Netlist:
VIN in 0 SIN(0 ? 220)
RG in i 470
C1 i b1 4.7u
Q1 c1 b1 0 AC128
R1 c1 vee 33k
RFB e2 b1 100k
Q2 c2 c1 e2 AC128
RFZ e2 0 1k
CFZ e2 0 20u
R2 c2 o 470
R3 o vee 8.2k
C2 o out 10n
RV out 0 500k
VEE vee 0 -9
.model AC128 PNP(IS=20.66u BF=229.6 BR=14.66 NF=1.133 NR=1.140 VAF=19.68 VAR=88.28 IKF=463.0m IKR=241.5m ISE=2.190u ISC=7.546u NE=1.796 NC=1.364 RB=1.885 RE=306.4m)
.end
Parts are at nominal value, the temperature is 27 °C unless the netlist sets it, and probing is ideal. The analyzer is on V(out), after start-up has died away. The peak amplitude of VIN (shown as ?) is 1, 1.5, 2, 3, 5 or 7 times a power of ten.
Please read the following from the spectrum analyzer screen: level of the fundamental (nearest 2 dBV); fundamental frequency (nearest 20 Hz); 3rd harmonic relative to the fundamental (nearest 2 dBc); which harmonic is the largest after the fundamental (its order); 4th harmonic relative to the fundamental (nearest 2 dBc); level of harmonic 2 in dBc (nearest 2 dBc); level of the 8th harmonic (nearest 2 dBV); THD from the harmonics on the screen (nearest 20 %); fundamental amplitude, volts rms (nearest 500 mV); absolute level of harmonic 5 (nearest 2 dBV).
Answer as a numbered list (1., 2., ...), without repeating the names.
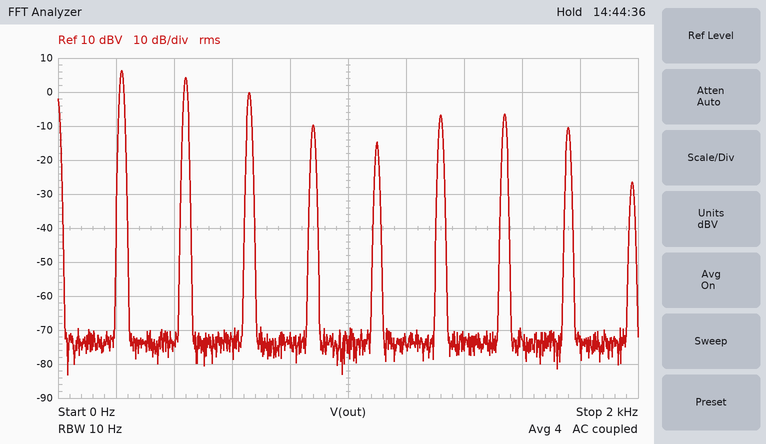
1. 6 dBV
2. 220 Hz
3. -6 dBc
4. 2
5. -16 dBc
6. -2 dBc
7. -10 dBV
8. 100 %
9. 2.0 V
10. -14 dBV
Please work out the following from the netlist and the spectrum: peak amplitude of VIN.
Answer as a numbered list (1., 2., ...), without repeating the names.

1. 500 mV
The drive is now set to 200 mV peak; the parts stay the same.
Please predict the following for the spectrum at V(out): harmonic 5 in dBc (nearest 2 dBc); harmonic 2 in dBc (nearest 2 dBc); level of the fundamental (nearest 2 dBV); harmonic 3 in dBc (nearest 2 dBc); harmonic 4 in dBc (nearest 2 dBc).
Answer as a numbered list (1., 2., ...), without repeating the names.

1. -12 dBc
2. -4 dBc
3. 8 dBV
4. -14 dBc
5. -18 dBc
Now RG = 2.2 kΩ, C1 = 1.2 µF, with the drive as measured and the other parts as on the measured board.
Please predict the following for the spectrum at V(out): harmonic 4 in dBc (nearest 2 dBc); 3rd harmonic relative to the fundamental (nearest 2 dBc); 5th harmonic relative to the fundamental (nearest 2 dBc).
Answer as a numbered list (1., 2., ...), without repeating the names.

1. -14 dBc
2. -22 dBc
3. -12 dBc
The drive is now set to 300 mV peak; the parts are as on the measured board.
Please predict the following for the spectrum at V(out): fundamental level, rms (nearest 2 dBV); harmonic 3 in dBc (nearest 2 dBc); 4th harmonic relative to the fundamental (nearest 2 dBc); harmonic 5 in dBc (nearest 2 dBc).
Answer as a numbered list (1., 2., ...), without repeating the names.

1. 8 dBV
2. -10 dBc
3. -44 dBc
4. -14 dBc
